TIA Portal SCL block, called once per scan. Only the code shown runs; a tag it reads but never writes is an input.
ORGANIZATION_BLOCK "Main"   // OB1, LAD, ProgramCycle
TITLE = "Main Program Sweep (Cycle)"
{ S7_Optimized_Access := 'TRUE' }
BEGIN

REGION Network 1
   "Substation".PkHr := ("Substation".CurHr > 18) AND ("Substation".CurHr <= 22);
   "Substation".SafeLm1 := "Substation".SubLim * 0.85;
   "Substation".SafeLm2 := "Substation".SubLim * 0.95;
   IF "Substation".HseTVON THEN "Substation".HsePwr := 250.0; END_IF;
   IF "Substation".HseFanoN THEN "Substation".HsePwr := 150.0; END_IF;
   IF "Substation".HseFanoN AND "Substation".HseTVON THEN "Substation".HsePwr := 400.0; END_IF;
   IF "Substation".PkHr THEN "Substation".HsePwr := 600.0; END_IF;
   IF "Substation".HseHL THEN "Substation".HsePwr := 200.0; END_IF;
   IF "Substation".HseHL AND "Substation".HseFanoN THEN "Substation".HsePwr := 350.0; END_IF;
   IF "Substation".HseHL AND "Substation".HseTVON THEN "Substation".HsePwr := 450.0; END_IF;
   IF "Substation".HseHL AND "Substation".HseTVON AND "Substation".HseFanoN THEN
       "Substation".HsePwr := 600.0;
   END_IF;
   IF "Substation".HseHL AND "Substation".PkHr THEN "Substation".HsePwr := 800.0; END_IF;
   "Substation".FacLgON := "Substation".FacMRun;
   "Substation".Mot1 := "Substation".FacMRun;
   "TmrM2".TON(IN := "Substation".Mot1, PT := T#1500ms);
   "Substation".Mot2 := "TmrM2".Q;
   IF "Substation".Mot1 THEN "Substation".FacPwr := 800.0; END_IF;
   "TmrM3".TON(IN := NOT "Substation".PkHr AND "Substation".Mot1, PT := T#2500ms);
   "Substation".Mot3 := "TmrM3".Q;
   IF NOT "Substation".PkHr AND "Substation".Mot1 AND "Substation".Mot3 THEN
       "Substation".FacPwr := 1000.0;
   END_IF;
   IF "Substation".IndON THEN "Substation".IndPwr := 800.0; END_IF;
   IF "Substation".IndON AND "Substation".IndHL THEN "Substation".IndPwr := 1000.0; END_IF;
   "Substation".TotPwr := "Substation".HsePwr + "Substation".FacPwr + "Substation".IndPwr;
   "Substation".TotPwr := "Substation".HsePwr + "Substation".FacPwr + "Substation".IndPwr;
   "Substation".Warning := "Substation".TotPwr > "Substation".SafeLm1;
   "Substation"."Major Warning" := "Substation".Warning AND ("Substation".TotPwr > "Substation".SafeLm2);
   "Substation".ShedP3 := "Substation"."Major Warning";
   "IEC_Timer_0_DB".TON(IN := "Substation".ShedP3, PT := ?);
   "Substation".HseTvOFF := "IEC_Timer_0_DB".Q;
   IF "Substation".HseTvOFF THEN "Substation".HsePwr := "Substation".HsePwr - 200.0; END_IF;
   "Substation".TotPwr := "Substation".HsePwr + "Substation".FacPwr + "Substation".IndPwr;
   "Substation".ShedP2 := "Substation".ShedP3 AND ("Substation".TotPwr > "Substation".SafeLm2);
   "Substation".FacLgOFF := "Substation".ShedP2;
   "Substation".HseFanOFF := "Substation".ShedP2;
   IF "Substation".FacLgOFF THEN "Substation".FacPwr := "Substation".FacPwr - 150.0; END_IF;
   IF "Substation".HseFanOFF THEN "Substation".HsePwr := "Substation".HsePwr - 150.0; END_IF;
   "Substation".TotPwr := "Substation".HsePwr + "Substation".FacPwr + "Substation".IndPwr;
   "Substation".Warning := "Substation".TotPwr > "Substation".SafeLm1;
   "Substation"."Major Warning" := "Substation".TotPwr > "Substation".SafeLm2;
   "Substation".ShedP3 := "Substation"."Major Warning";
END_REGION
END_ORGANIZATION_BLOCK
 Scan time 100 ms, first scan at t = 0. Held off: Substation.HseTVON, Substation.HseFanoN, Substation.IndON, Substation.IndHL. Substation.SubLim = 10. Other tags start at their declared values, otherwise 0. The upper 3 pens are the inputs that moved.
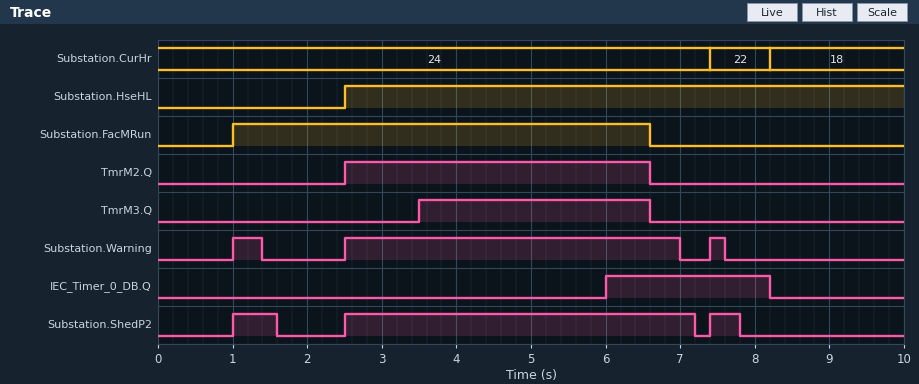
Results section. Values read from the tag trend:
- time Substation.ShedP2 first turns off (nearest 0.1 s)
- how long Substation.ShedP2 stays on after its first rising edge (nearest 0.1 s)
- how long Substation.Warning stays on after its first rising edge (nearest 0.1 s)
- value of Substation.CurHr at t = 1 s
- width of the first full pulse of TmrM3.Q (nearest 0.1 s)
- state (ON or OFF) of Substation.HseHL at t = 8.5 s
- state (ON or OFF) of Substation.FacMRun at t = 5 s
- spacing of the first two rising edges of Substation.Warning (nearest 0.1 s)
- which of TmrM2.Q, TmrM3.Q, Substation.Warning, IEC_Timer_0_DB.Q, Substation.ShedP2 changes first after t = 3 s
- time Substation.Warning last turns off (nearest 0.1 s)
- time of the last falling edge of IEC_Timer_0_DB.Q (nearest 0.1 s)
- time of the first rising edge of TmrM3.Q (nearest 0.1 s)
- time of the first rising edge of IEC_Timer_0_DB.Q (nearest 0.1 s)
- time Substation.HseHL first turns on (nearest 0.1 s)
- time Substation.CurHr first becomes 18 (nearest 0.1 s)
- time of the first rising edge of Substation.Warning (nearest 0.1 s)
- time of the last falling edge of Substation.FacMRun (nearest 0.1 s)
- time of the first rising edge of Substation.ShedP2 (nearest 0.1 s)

1.6 s
0.6 s
0.4 s
24
3.1 s
ON
ON
1.5 s
TmrM3.Q
7.6 s
8.2 s
3.5 s
6.0 s
2.5 s
8.2 s
1.0 s
6.6 s
1.0 s
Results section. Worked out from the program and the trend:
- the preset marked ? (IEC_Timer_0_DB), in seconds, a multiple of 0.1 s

3.5 s
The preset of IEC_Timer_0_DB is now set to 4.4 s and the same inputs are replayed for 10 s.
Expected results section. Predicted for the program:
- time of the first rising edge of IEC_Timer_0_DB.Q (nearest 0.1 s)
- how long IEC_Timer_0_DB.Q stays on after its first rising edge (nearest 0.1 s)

6.9 s
1.3 s
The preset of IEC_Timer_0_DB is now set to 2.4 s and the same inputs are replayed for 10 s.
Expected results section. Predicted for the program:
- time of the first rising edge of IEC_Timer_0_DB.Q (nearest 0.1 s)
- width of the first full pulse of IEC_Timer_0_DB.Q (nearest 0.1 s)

4.9 s
3.3 s
